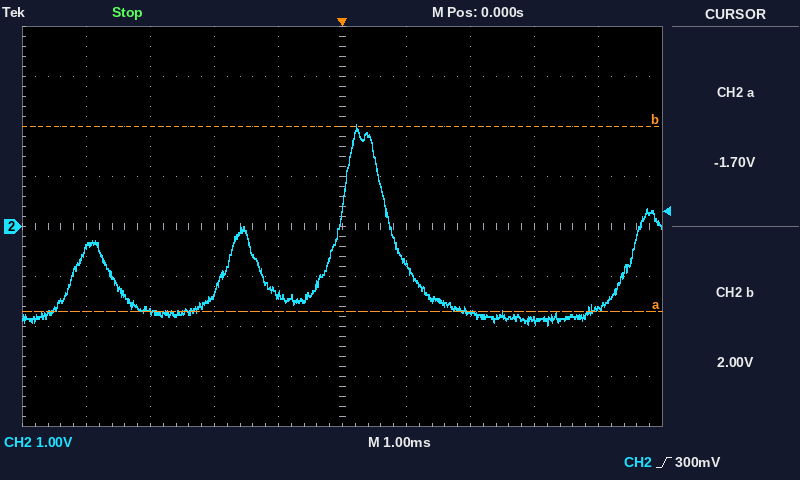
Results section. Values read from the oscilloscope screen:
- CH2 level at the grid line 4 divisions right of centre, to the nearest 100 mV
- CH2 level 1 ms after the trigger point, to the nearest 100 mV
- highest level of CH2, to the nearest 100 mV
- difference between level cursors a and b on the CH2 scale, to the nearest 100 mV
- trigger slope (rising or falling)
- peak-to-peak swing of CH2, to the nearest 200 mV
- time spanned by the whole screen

-1.6 V
-700 mV
2.0 V
3.7 V
rising
4.0 V
10 ms
